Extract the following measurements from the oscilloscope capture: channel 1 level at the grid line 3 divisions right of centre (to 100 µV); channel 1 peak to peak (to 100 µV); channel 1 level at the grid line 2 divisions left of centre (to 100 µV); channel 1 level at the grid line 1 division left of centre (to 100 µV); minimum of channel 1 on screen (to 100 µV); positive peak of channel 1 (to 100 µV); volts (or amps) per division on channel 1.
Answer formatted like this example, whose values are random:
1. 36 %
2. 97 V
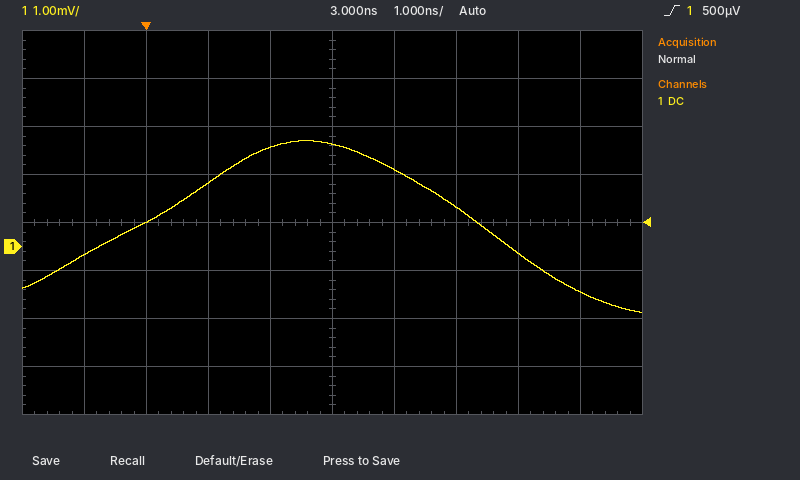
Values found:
1. -100 µV
2. 3.6 mV
3. 1.3 mV
4. 2.1 mV
5. -1.4 mV
6. 2.2 mV
7. 1 mV
